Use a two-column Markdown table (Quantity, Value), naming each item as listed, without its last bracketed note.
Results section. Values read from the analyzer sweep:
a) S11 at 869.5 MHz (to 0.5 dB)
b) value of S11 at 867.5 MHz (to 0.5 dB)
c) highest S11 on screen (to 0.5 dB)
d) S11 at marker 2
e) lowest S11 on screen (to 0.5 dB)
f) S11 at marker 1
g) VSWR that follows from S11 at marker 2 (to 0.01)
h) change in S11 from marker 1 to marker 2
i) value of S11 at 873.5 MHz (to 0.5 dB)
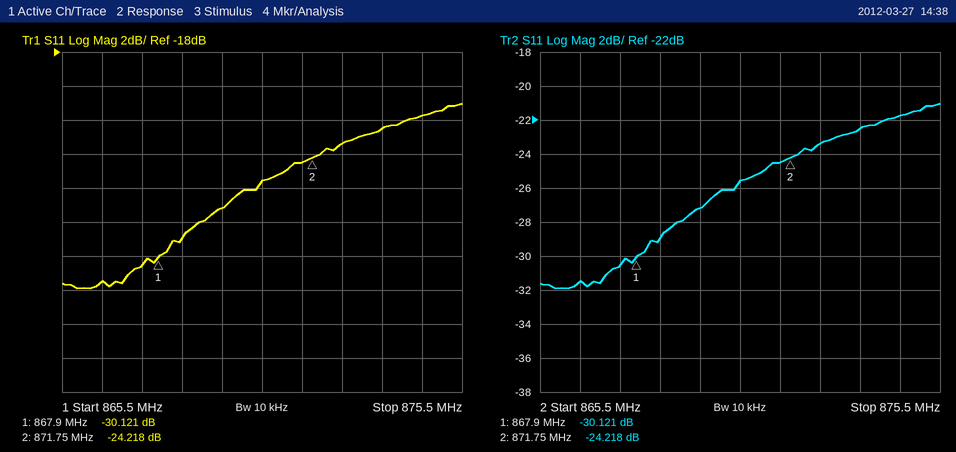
| Quantity | Value |
|---|---|
| S11 at 869.5 MHz | -27.0 dB |
| value of S11 at 867.5 MHz | -30.5 dB |
| highest S11 on screen | -21.0 dB |
| S11 at marker 2 | -24.218 dB |
| lowest S11 on screen | -32.0 dB |
| S11 at marker 1 | -30.121 dB |
| VSWR that follows from S11 at marker 2 | 1.13 |
| change in S11 from marker 1 to marker 2 | 5.903 dB |
| value of S11 at 873.5 MHz | -22.5 dB |
